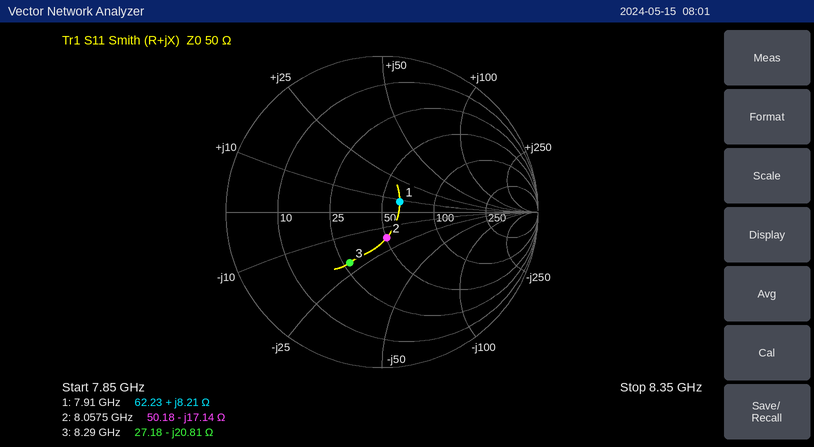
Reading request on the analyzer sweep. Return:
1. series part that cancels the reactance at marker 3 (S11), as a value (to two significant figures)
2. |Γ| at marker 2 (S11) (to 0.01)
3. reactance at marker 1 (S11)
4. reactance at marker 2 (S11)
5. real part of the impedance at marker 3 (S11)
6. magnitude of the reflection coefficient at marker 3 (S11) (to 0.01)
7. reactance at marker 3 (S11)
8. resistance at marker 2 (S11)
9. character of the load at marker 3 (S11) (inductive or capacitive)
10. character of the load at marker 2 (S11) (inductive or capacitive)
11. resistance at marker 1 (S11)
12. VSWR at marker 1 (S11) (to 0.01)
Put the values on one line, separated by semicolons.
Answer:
400 pH; 0.17; +8.21 Ω; -17.14 Ω; 27.18 Ω; 0.39; -20.81 Ω; 50.18 Ω; capacitive; capacitive; 62.23 Ω; 1.30
